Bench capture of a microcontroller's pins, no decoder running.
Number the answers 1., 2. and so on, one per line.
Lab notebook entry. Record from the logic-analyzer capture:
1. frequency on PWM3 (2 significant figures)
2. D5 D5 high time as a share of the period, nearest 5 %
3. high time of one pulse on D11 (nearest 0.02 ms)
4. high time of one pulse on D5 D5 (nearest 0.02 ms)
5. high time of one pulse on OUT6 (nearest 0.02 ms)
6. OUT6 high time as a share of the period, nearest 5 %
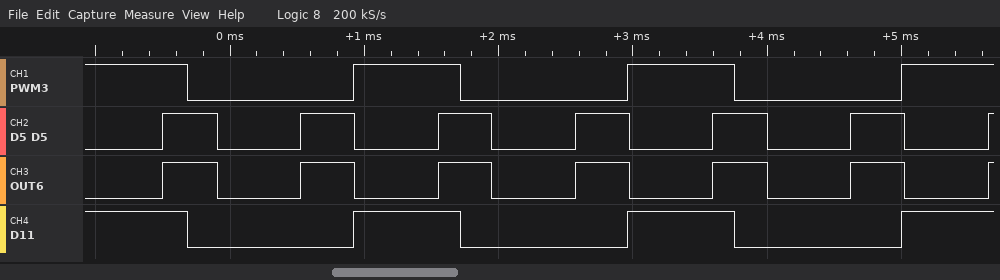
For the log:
1. 490 Hz
2. 40 %
3. 0.80 ms
4. 0.40 ms
5. 0.40 ms
6. 40 %
